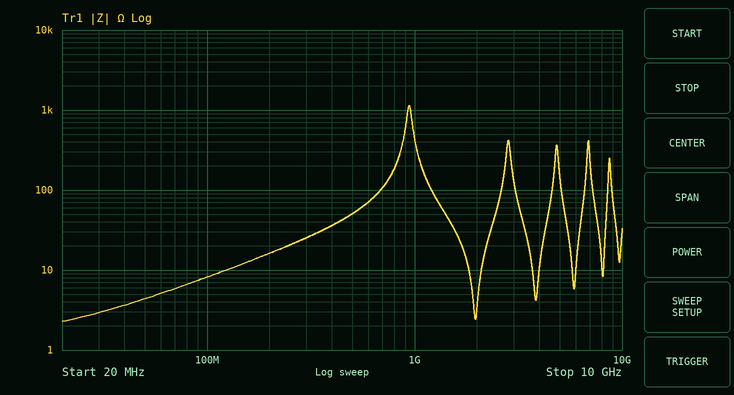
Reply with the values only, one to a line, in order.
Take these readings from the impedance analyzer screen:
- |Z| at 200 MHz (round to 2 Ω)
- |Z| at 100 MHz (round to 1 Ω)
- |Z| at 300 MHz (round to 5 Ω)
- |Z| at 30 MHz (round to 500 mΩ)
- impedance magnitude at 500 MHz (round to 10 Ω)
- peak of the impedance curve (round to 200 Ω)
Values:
16 Ω
8 Ω
25 Ω
3.0 Ω
50 Ω
1.2 kΩ
